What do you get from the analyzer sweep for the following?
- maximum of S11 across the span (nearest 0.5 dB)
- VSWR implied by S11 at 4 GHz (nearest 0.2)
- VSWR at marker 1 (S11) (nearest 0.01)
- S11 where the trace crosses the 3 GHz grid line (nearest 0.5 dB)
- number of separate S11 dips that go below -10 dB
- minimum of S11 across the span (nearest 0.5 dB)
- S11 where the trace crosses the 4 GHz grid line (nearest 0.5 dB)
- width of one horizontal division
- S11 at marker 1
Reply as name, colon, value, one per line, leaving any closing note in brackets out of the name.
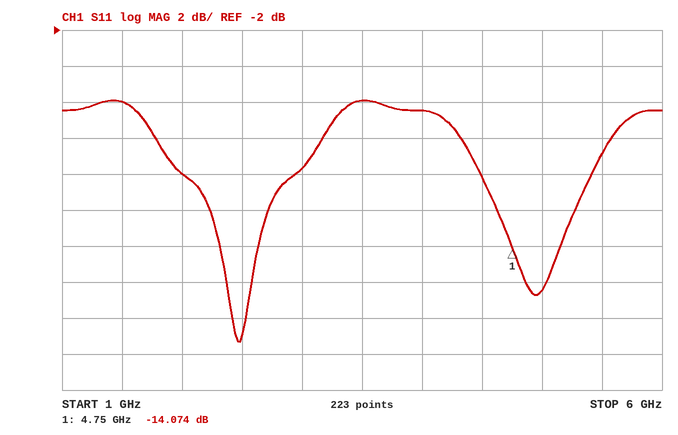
maximum of S11 across the span: -6.0 dB
VSWR implied by S11 at 4 GHz: 2.8
VSWR at marker 1 (S11): 1.49
S11 where the trace crosses the 3 GHz grid line: -9.5 dB
number of separate S11 dips that go below -10 dB: 2
minimum of S11 across the span: -19.5 dB
S11 where the trace crosses the 4 GHz grid line: -6.5 dB
width of one horizontal division: 500 MHz
S11 at marker 1: -14.074 dB
